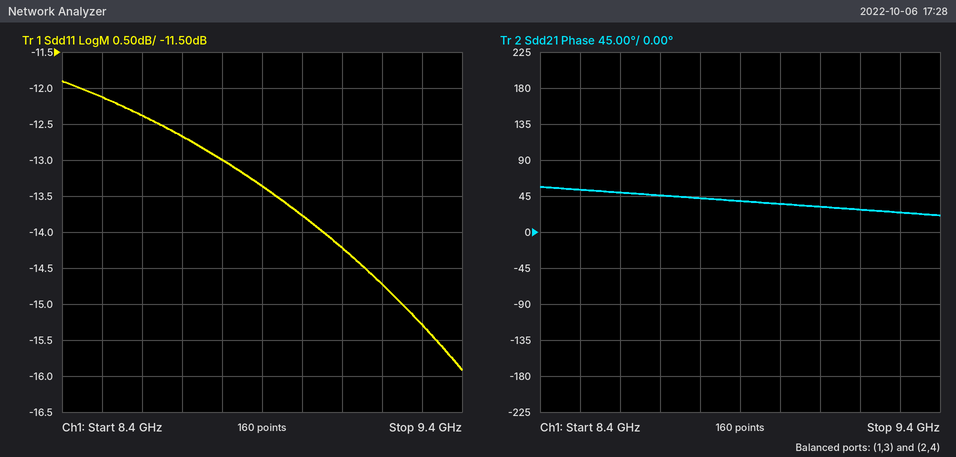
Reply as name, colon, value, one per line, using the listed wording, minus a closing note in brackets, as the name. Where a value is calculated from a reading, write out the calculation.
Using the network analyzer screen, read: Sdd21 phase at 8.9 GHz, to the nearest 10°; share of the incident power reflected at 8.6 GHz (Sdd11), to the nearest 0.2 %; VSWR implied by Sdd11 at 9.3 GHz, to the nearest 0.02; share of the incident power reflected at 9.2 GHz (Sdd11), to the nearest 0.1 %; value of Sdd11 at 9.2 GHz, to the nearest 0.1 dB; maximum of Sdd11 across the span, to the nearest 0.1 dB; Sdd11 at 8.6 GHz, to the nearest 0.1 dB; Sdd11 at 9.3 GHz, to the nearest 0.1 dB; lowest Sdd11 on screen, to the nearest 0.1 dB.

Sdd21 phase at 8.9 GHz, to the nearest 10°: 40°
share of the incident power reflected at 8.6 GHz (Sdd11), to the nearest 0.2 %: 10^(-12.4/10) ≈ 5.8 %
VSWR implied by Sdd11 at 9.3 GHz, to the nearest 0.02: |Γ| = 10^(-15.3/20) = 0.1718; VSWR = (1 + 0.1718)/(1 − 0.1718) ≈ 1.41, so 1.42 to the nearest 0.02
share of the incident power reflected at 9.2 GHz (Sdd11), to the nearest 0.1 %: 10^(-14.7/10) ≈ 3.4 %
value of Sdd11 at 9.2 GHz, to the nearest 0.1 dB: -14.7 dB
maximum of Sdd11 across the span, to the nearest 0.1 dB: -11.9 dB
Sdd11 at 8.6 GHz, to the nearest 0.1 dB: -12.4 dB
Sdd11 at 9.3 GHz, to the nearest 0.1 dB: -15.3 dB
lowest Sdd11 on screen, to the nearest 0.1 dB: -15.9 dB
